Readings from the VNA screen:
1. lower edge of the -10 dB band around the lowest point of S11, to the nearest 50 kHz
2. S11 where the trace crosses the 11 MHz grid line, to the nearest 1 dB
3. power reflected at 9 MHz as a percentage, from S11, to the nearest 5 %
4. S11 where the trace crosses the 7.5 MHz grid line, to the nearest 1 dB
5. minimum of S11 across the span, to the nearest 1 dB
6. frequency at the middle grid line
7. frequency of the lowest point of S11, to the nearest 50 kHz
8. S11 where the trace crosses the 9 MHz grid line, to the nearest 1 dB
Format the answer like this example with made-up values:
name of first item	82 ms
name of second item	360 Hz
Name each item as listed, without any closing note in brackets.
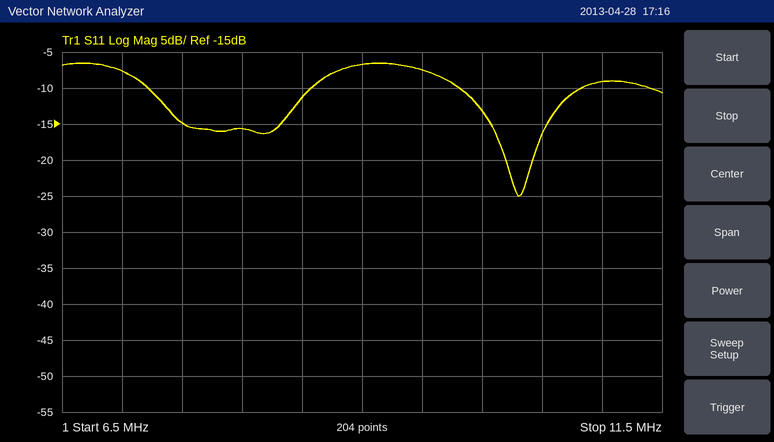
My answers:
lower edge of the -10 dB band around the lowest point of S11, to the nearest 50 kHz	9.80 MHz
S11 where the trace crosses the 11 MHz grid line, to the nearest 1 dB	-9 dB
power reflected at 9 MHz as a percentage, from S11, to the nearest 5 %	20 %
S11 where the trace crosses the 7.5 MHz grid line, to the nearest 1 dB	-15 dB
minimum of S11 across the span, to the nearest 1 dB	-25 dB
frequency at the middle grid line	9 MHz
frequency of the lowest point of S11, to the nearest 50 kHz	10.30 MHz
S11 where the trace crosses the 9 MHz grid line, to the nearest 1 dB	-7 dB
